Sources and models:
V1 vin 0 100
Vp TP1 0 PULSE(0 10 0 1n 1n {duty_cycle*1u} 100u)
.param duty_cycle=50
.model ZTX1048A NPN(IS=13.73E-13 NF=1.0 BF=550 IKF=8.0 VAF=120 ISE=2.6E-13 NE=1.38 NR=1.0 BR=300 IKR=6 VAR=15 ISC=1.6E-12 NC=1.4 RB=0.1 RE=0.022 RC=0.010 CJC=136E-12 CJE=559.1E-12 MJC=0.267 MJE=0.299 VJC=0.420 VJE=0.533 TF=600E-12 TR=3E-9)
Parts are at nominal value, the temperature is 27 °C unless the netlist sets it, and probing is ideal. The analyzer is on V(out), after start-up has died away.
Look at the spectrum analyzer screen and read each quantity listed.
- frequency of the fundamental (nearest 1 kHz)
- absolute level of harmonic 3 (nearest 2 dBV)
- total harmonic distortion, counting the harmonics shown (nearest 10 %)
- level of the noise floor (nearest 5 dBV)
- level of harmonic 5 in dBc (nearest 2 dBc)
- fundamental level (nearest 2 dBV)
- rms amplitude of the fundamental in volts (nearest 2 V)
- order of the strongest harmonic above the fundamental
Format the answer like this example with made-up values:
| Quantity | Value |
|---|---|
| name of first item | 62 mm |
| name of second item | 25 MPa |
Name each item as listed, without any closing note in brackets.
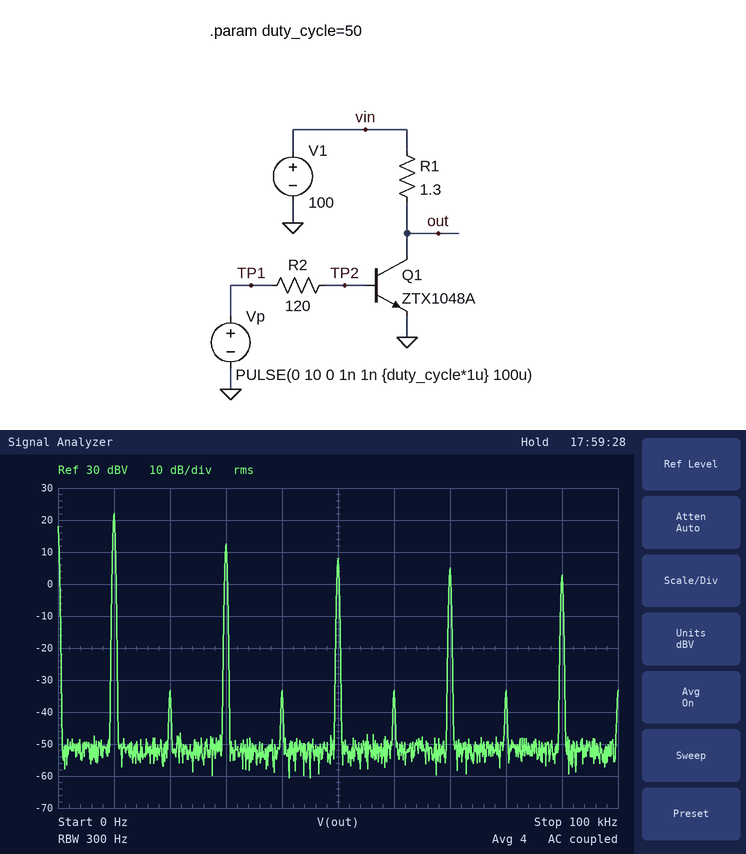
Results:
| Quantity | Value |
|---|---|
| frequency of the fundamental | 10 kHz |
| absolute level of harmonic 3 | 12 dBV |
| total harmonic distortion, counting the harmonics shown | 40 % |
| level of the noise floor | -50 dBV |
| level of harmonic 5 in dBc | -14 dBc |
| fundamental level | 22 dBV |
| rms amplitude of the fundamental in volts | 12 V |
| order of the strongest harmonic above the fundamental | 3 |
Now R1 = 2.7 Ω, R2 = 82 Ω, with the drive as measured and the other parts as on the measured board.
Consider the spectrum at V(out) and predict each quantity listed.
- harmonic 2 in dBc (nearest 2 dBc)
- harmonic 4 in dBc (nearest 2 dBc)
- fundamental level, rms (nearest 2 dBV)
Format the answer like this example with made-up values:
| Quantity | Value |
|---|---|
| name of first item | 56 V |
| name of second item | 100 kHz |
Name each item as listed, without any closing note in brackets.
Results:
| Quantity | Value |
|---|---|
| harmonic 2 in dBc | -54 dBc |
| harmonic 4 in dBc | -54 dBc |
| fundamental level, rms | 28 dBV |
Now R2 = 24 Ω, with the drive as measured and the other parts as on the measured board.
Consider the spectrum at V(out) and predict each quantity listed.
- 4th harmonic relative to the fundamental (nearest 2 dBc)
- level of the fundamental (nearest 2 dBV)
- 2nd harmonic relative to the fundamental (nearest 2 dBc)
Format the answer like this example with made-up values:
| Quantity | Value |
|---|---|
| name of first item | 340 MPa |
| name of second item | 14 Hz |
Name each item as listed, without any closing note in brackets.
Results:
| Quantity | Value |
|---|---|
| 4th harmonic relative to the fundamental | -58 dBc |
| level of the fundamental | 28 dBV |
| 2nd harmonic relative to the fundamental | -58 dBc |
